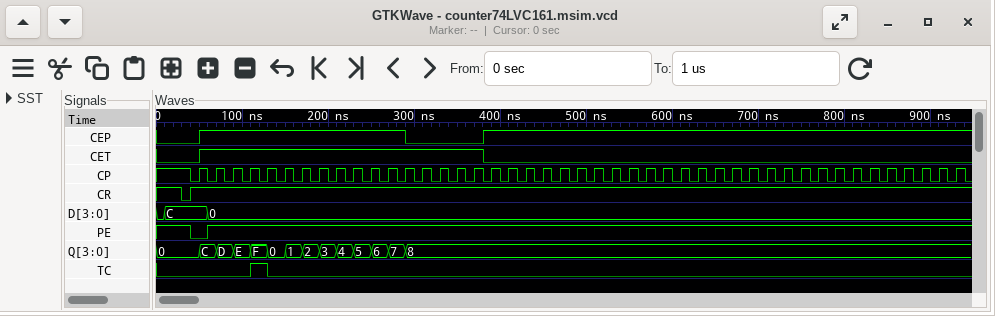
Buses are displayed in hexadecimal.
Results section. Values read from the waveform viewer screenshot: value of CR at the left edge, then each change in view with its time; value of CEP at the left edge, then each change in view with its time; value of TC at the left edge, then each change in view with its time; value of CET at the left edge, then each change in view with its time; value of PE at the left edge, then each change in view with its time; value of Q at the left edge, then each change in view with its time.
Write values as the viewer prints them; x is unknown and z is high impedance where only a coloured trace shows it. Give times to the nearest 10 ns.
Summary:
1, 0 at 30 ns, 1 at 40 ns
0, 1 at 50 ns, 0 at 290 ns, 1 at 380 ns
0, 1 at 110 ns, 0 at 130 ns
0, 1 at 50 ns, 0 at 380 ns
1, 0 at 40 ns, 1 at 60 ns
0, C at 50 ns, D at 70 ns, E at 90 ns, F at 110 ns, 0 at 130 ns, 1 at 150 ns, 2 at 170 ns, 3 at 190 ns, 4 at 210 ns, 5 at 230 ns, 6 at 250 ns, 7 at 270 ns, 8 at 290 ns
